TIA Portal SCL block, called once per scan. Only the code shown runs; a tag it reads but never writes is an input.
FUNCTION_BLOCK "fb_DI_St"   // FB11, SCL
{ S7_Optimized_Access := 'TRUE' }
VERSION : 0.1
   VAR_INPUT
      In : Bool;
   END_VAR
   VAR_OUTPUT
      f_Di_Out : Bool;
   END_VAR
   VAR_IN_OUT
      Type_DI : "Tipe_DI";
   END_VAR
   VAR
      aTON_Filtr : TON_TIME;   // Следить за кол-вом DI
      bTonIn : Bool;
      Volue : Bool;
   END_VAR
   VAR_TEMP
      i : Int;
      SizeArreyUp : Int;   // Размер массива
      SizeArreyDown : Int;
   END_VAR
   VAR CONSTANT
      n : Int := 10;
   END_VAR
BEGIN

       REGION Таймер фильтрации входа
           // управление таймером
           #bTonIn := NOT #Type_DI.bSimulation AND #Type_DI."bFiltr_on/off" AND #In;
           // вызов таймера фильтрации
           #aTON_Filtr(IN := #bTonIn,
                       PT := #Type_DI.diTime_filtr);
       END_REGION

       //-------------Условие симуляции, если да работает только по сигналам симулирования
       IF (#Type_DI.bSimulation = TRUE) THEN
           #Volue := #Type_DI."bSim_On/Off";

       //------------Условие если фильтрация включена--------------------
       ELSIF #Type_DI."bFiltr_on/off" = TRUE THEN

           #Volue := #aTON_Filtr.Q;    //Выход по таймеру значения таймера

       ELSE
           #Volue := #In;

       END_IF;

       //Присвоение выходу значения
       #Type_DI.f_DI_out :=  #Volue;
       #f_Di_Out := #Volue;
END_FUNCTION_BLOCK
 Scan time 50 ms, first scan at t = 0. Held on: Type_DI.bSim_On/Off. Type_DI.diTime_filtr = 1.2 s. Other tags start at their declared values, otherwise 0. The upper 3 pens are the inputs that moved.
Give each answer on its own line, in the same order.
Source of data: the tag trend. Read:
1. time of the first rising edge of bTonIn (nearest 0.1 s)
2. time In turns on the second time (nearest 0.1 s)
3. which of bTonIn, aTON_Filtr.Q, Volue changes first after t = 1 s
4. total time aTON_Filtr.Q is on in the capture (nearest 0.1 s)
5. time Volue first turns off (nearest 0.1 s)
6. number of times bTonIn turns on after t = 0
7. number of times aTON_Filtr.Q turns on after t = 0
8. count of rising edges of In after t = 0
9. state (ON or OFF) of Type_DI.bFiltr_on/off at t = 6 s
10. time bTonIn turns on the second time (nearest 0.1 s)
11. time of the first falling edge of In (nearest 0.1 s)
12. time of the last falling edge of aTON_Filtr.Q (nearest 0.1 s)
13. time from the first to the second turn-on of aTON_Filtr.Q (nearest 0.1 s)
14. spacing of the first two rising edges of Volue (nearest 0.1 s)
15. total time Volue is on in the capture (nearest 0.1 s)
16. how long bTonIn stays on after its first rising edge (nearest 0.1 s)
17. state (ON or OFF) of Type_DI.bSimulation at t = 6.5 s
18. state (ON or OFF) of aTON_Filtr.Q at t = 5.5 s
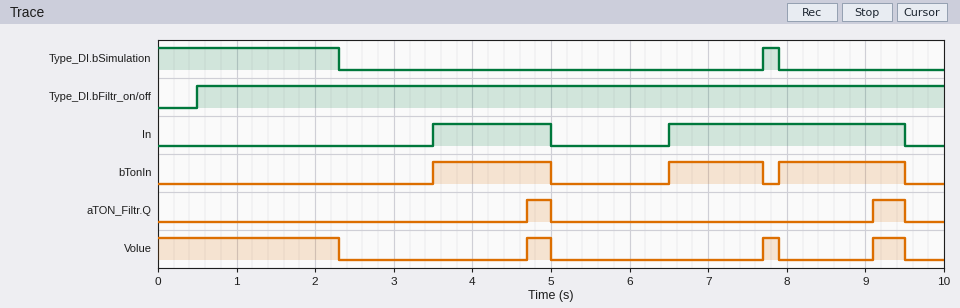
3.5 s
6.5 s
Volue
0.7 s
2.3 s
3
2
2
ON
6.5 s
5.0 s
9.5 s
4.4 s
3.0 s
3.2 s
1.5 s
OFF
OFF
